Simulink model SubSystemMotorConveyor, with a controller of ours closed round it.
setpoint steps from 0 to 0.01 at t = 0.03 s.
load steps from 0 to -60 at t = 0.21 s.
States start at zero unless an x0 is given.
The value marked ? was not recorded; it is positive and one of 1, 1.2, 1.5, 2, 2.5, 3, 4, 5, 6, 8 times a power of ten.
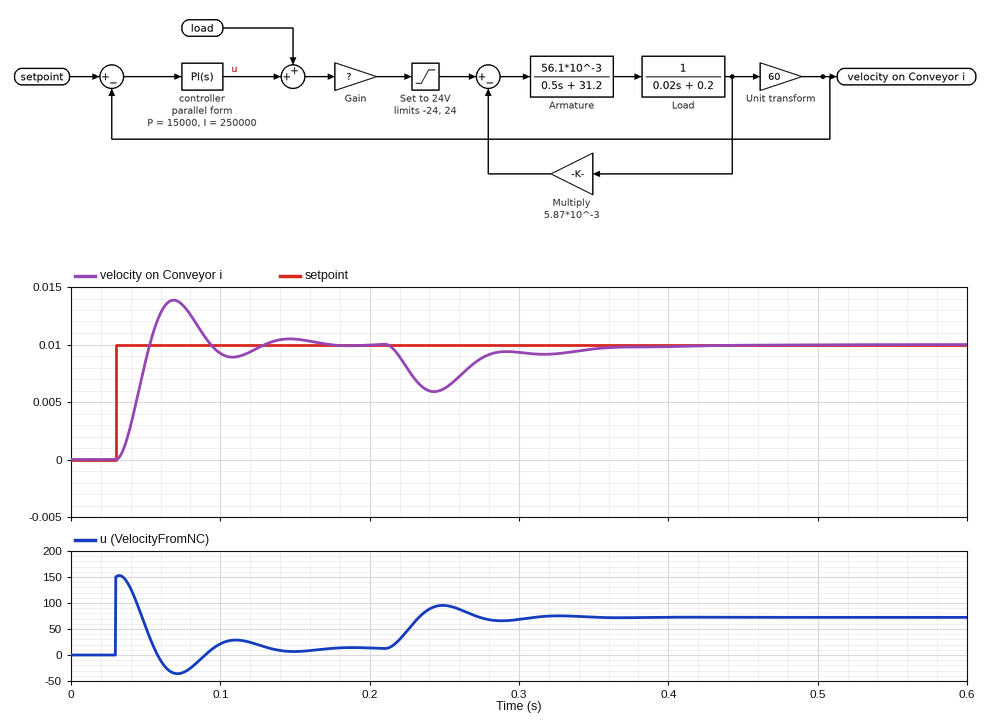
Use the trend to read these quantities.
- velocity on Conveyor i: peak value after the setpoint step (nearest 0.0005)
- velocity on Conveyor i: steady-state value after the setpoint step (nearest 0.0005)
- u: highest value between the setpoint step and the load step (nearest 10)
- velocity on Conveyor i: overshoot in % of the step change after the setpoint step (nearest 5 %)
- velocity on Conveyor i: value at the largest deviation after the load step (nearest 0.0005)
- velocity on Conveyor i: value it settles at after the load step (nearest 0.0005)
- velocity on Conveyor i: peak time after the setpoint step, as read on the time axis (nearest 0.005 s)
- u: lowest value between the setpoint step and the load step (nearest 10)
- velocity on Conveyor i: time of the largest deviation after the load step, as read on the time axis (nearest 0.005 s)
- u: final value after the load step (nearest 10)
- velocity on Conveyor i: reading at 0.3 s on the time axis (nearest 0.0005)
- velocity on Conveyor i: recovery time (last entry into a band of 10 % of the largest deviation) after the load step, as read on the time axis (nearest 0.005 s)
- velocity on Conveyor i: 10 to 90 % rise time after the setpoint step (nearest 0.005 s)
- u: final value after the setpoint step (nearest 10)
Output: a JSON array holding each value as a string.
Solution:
["0.0140", "0.0100", "150", "40 %", "0.0060", "0.0100", "0.070 s", "-40", "0.245 s", "70", "0.0095", "0.350 s", "0.015 s", "10"]
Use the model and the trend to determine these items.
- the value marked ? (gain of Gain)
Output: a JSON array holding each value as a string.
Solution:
["0.0015"]
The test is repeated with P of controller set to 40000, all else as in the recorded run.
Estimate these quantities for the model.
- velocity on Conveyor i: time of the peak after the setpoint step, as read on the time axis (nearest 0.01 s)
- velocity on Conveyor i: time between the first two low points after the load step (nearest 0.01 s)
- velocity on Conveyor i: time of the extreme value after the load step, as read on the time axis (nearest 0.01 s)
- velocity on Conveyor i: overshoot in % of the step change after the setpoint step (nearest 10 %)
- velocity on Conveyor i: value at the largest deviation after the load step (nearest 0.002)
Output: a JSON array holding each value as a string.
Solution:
["0.05 s", "0.04 s", "0.23 s", "50 %", "0.008"]
